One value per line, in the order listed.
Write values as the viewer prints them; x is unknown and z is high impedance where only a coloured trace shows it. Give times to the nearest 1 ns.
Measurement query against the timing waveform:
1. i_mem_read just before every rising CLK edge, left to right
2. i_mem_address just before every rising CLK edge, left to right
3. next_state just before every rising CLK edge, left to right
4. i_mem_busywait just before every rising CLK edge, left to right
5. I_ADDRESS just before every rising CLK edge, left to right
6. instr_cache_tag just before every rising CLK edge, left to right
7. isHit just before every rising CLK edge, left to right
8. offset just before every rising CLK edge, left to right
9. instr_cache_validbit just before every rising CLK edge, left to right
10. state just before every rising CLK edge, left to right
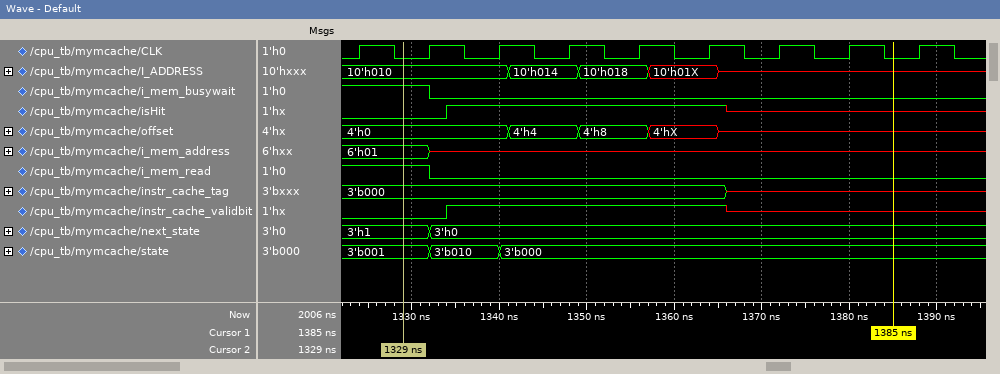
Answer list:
1 1 0 0 0 0 0 0 0
6'h01, 6'h01, x, x, x, x, x, x, x
3'h1, 3'h1, 3'h0, 3'h0, 3'h0, 3'h0, 3'h0, 3'h0, 3'h0
1 1 0 0 0 0 0 0 0
10'h010, 10'h010, 10'h010, 10'h014, 10'h018, 10'h01X, x, x, x
3'b000, 3'b000, 3'b000, 3'b000, 3'b000, 3'b000, x, x, x
0 0 1 1 1 1 x x x
4'h0, 4'h0, 4'h0, 4'h4, 4'h8, 4'hX, x, x, x
0 0 1 1 1 1 x x x
3'b001, 3'b001, 3'b010, 3'b000, 3'b000, 3'b000, 3'b000, 3'b000, 3'b000
